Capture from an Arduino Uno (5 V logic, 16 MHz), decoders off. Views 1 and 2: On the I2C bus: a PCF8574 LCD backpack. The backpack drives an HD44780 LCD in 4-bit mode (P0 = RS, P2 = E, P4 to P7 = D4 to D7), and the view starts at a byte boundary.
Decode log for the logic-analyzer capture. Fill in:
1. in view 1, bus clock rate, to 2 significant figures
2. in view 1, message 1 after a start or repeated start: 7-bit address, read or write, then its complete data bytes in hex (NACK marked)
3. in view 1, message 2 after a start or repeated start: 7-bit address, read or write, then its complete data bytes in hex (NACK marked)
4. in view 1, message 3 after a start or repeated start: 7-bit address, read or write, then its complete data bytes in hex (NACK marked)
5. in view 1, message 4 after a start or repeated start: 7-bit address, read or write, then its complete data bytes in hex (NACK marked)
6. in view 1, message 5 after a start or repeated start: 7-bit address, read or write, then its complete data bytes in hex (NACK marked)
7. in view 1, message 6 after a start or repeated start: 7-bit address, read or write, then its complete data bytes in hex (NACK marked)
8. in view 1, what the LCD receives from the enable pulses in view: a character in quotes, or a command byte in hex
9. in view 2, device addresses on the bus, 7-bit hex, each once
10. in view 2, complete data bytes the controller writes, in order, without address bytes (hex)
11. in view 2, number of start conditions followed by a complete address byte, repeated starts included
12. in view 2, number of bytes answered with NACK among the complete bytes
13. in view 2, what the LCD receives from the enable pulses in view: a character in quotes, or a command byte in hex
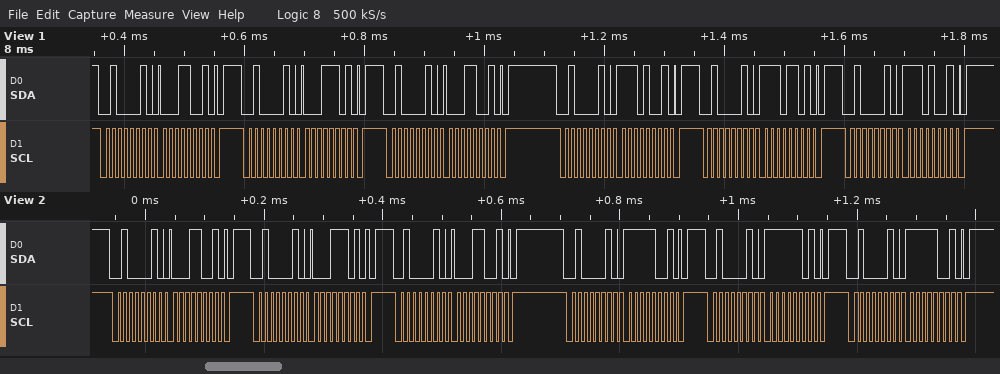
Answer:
100 kHz
0x21 write: 19
0x21 write: 1D
0x21 write: 19
0x21 write: E9
0x21 write: ED
0x21 write: E9
data 0x1E
0x21
19 1D 19 F9 FD F9
6
0
data 0x1F
